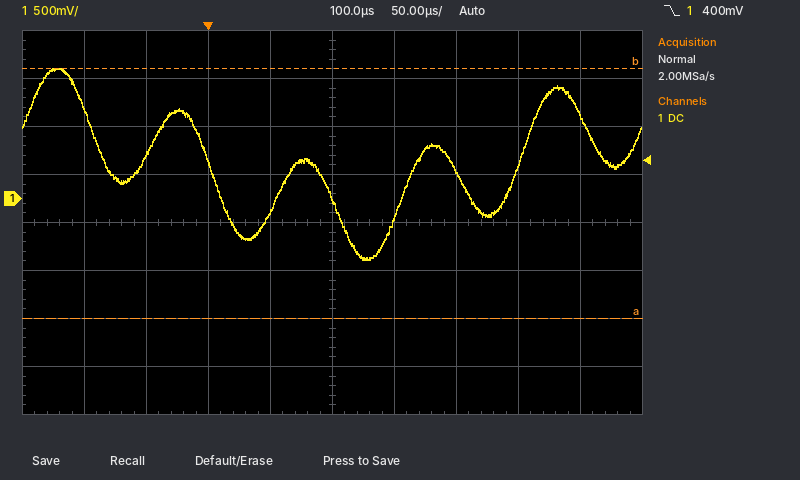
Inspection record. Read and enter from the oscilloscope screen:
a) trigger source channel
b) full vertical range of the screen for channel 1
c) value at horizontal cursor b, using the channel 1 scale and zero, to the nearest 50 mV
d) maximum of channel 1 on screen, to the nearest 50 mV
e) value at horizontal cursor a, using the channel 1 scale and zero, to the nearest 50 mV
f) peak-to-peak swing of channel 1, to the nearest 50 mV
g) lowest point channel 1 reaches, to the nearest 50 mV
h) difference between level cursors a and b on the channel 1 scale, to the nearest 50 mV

channel 1
4 V
1.35 V
1.35 V
-1.25 V
2.00 V
-650 mV
2.60 V
